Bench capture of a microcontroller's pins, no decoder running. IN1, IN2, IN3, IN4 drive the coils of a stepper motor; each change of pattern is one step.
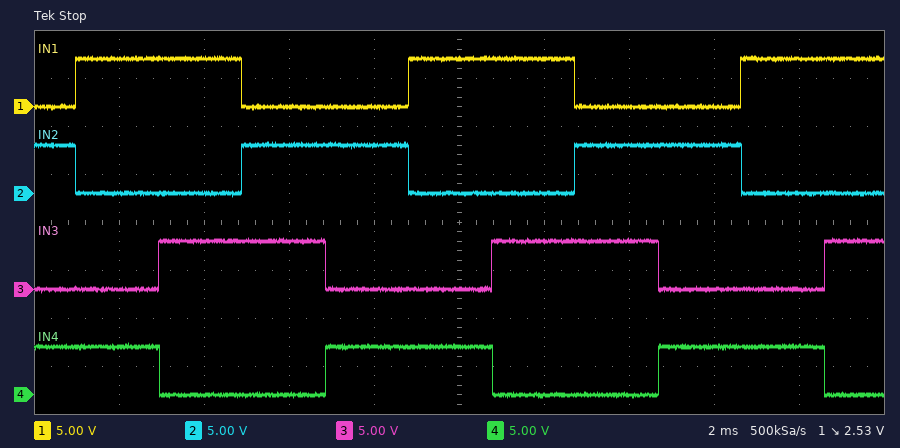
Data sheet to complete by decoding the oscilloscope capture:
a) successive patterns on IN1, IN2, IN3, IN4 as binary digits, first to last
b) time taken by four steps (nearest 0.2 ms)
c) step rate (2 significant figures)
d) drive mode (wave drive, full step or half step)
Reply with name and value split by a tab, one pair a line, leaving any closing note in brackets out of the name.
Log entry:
successive patterns on IN1, IN2, IN3, IN4 as binary digits, first to last	0101 1001 1010 0110 0101 1001 1010 0110 0101 1001 1010
time taken by four steps	7.8 ms
step rate	510 steps/s
drive mode	full step
